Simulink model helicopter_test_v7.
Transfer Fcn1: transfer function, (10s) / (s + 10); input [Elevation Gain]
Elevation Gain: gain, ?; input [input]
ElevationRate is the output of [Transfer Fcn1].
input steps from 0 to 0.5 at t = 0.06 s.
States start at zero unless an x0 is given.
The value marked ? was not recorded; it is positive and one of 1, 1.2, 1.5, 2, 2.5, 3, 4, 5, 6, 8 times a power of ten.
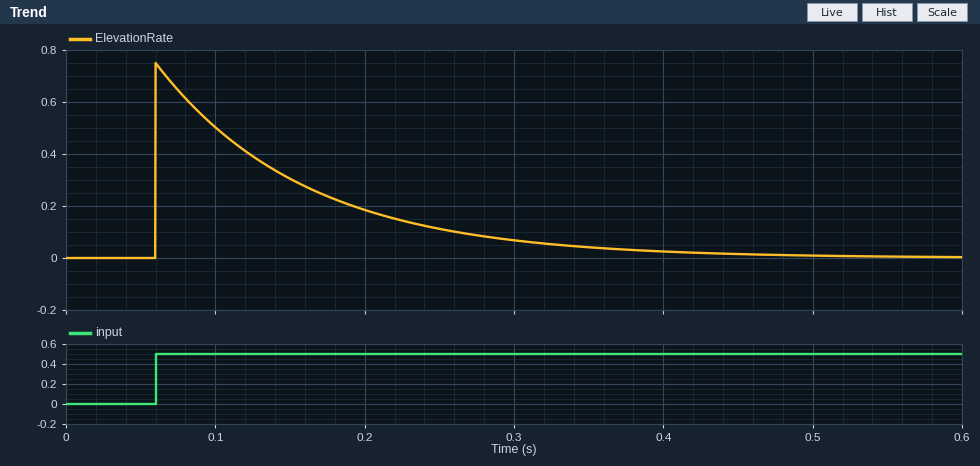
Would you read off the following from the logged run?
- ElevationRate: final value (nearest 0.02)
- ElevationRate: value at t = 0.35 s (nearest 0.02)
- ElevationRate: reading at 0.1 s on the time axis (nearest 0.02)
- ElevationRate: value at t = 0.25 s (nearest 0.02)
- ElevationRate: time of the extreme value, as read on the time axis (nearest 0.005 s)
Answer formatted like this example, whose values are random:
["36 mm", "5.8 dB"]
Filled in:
["0.00", "0.04", "0.50", "0.12", "0.060 s"]
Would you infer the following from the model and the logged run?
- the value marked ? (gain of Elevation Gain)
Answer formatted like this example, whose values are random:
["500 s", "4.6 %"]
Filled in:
["0.15"]
